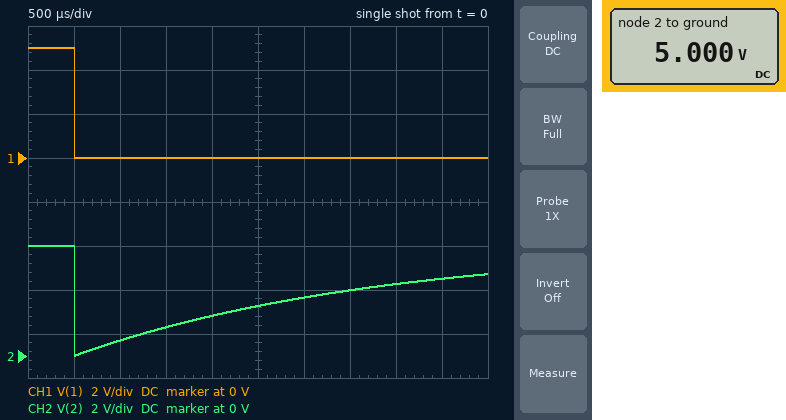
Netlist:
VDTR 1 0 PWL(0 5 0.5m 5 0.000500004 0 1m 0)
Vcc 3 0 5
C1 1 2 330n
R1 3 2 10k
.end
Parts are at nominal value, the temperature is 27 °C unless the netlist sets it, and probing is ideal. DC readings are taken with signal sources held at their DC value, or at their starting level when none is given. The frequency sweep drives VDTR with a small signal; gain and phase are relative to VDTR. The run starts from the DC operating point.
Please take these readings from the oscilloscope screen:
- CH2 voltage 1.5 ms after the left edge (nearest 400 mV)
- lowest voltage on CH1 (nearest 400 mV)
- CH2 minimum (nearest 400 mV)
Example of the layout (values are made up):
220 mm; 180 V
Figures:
1.2 V; 0 V; 0 V
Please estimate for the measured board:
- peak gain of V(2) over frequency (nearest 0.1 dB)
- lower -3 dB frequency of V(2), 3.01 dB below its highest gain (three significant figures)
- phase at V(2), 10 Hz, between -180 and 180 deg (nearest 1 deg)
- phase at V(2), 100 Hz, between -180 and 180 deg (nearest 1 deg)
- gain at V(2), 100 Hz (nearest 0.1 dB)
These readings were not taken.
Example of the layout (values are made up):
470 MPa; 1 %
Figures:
0 dB; 48.2 Hz; 78 deg; 26 deg; -0.9 dB
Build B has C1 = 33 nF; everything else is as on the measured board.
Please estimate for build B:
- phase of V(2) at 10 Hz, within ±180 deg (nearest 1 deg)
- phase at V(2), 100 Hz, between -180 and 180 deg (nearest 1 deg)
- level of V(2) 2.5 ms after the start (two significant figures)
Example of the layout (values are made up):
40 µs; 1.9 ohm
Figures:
89 deg; 78 deg; 5.0 V
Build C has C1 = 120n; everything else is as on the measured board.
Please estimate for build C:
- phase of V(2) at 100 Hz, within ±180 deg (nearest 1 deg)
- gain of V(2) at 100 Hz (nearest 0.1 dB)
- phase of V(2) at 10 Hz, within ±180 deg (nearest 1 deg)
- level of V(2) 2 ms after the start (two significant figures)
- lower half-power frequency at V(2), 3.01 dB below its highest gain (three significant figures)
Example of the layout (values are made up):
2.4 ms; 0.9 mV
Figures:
53 deg; -4.4 dB; 86 deg; 3.6 V; 133 Hz
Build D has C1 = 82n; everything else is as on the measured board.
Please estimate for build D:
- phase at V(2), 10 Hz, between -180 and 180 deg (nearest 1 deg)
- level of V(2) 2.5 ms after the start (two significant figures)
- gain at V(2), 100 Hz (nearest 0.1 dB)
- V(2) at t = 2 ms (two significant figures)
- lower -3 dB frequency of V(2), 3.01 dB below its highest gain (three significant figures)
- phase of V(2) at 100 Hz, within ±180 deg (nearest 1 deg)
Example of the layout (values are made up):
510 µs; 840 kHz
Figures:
87 deg; 4.6 V; -6.8 dB; 4.2 V; 194 Hz; 63 deg
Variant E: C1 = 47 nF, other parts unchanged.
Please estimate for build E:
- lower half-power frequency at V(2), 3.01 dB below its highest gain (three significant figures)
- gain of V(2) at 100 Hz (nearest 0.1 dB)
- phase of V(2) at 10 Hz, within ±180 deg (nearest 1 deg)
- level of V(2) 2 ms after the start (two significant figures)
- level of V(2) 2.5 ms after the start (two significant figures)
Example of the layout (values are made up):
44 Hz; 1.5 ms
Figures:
339 Hz; -11.0 dB; 88 deg; 4.8 V; 4.9 V
